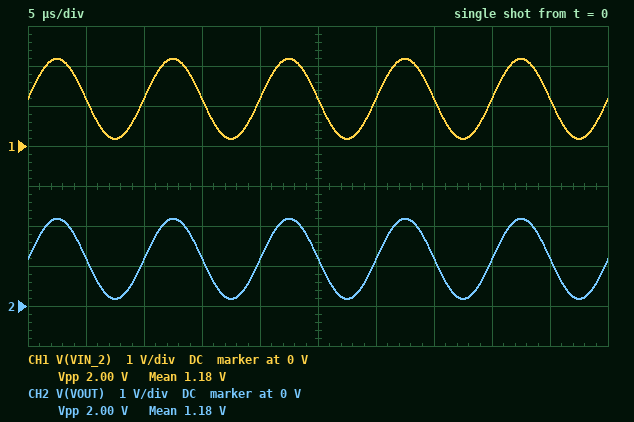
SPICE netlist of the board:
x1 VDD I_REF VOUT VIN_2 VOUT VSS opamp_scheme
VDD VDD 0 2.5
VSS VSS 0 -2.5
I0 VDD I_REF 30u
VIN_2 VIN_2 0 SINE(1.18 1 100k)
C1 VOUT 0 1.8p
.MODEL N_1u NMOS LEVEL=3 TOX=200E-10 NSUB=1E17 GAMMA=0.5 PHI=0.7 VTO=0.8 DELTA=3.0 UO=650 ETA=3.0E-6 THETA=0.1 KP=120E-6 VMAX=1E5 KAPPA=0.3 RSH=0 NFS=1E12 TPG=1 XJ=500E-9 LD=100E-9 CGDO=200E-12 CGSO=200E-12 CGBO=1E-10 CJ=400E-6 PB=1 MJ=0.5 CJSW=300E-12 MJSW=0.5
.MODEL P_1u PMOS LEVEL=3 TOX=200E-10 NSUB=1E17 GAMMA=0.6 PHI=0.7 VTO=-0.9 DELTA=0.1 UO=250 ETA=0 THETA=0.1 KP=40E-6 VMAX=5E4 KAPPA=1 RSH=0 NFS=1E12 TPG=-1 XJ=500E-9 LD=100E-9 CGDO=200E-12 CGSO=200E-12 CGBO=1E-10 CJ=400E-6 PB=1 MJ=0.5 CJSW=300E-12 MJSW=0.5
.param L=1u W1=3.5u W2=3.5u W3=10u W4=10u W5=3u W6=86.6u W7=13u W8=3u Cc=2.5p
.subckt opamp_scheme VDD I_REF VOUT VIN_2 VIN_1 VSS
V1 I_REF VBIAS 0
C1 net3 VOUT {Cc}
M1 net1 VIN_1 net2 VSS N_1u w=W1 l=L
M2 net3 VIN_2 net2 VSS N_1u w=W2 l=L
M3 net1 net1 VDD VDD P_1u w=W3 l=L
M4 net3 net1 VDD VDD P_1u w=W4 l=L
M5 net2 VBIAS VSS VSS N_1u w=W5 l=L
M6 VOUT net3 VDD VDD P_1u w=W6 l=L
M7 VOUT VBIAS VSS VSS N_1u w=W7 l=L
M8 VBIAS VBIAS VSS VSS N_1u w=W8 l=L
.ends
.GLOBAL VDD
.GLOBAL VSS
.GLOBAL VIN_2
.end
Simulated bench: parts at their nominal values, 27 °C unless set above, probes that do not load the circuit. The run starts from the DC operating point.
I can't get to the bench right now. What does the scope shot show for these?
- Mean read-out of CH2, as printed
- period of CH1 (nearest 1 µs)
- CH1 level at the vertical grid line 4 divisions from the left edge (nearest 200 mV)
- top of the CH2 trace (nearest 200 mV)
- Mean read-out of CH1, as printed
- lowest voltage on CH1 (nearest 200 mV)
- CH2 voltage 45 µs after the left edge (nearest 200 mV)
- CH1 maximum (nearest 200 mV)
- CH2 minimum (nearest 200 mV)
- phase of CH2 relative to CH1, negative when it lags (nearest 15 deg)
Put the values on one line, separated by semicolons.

1.18 V; 10 µs; 1.2 V; 2.2 V; 1.18 V; 200 mV; 1.2 V; 2.2 V; 200 mV; 0 deg
